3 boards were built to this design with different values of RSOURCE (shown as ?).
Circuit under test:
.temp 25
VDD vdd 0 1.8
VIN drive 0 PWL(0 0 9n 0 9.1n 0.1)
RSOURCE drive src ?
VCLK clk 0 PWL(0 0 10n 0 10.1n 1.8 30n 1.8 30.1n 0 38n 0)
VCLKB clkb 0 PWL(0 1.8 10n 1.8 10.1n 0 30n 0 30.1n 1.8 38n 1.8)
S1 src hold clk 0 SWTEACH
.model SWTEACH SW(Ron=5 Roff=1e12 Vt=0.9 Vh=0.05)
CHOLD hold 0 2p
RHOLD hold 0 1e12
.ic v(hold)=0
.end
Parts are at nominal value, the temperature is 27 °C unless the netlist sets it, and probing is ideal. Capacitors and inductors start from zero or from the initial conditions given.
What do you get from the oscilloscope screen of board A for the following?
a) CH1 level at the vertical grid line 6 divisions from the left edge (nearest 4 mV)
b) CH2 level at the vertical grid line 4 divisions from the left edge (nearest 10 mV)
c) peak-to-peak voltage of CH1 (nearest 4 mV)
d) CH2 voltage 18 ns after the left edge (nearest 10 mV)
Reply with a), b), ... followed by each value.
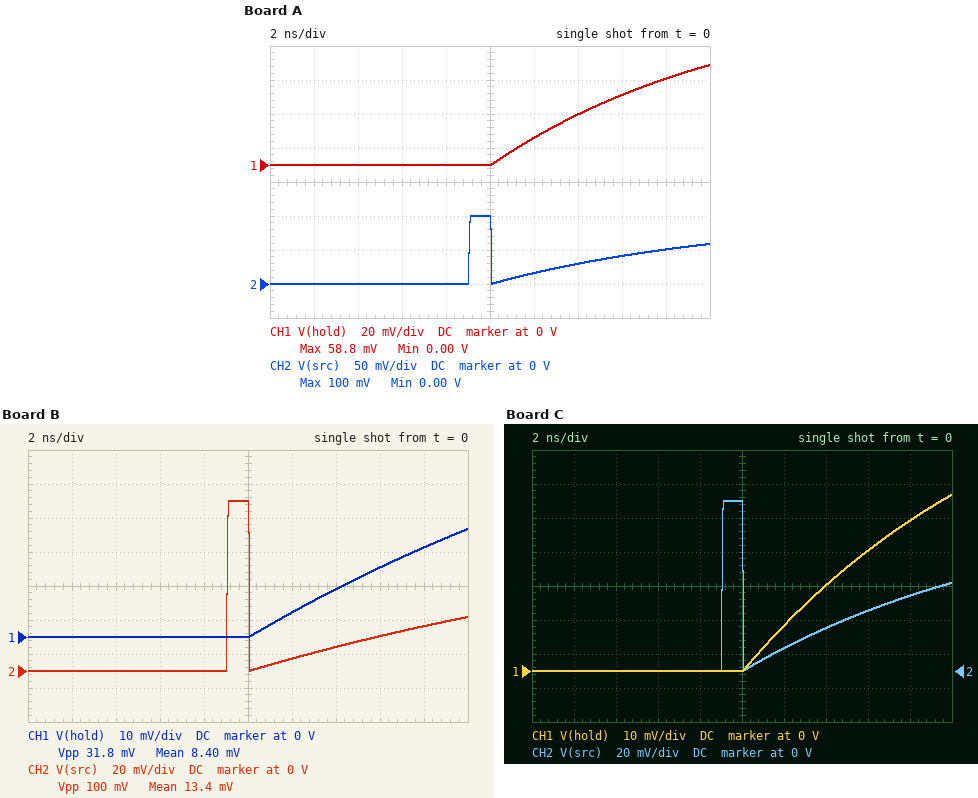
a) 16 mV
b) 0 V
c) 60 mV
d) 50 mV
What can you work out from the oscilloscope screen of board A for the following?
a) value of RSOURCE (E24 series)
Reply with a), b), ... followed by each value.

a) 5.6 kΩ
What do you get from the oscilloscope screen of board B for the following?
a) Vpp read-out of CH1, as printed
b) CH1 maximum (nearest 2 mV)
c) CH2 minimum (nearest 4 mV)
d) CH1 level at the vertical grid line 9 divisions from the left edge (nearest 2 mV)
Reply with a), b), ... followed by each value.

a) 31.8 mV
b) 32 mV
c) 0 V
d) 26 mV
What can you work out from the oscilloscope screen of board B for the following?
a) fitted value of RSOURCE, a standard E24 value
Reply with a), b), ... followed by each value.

a) 13 kΩ
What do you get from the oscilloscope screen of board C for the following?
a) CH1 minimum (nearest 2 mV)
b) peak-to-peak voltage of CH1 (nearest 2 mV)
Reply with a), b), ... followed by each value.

a) 0 V
b) 52 mV
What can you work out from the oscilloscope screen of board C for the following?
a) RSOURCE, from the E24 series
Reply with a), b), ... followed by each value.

a) 6.8 kΩ
